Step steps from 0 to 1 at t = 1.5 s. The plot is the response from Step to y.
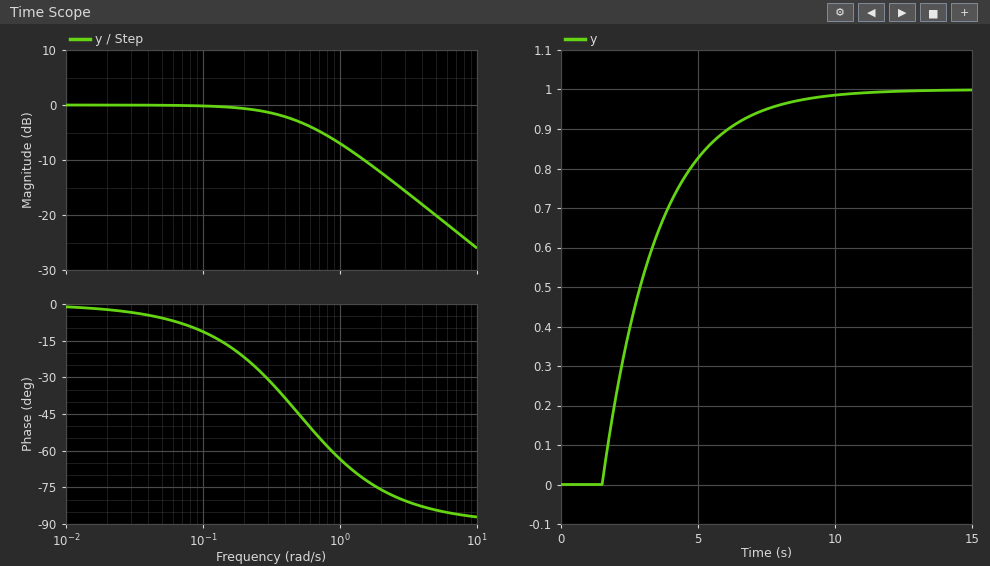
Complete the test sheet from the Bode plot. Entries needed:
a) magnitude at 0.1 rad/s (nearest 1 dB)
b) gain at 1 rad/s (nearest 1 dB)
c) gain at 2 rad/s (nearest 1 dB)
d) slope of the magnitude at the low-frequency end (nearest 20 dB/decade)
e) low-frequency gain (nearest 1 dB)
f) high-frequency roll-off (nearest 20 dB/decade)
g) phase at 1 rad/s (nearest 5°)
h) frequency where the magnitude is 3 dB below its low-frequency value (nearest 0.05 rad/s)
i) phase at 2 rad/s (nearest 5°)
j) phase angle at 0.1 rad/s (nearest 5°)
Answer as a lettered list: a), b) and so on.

a) 0 dB
b) -7 dB
c) -12 dB
d) 0 dB/decade
e) 0 dB
f) -20 dB/decade
g) -65°
h) 0.50 rad/s
i) -75°
j) -10°
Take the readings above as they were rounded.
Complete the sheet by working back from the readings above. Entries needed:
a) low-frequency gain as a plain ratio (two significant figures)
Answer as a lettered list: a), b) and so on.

a) 1.0
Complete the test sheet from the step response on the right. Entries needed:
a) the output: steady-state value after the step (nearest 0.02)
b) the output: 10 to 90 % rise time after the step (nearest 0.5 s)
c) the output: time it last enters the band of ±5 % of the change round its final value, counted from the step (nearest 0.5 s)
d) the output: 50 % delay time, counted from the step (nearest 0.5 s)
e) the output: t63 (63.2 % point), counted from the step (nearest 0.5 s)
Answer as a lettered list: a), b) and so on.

a) 1.00
b) 4.5 s
c) 6.0 s
d) 1.5 s
e) 2.0 s
